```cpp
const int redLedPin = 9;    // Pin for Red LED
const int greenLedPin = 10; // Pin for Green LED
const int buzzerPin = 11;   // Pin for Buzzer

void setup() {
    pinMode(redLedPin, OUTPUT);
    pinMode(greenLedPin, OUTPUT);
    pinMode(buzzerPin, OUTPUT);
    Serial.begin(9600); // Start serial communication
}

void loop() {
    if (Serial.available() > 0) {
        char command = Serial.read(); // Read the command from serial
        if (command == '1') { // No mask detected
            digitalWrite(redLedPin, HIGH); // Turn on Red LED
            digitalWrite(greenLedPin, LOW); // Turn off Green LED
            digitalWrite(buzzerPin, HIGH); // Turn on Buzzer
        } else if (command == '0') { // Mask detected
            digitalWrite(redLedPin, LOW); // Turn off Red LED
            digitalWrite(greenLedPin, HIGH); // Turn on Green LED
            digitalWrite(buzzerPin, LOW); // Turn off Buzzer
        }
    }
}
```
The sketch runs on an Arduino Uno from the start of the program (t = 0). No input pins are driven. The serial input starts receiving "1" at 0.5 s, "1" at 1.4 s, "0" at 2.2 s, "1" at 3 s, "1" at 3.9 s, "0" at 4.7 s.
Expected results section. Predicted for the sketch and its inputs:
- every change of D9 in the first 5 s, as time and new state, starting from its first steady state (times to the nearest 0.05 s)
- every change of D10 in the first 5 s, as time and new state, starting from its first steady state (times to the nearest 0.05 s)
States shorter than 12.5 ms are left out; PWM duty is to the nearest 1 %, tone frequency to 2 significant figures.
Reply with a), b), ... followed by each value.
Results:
a) 0 s low; 0.5 s high; 2.2 s low; 3 s high; 4.7 s low
b) 0 s low; 2.2 s high; 3 s low; 4.7 s high
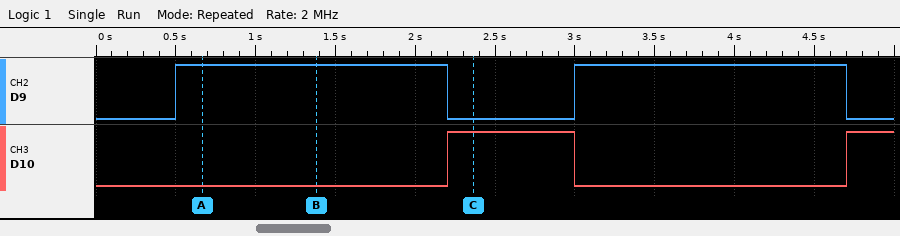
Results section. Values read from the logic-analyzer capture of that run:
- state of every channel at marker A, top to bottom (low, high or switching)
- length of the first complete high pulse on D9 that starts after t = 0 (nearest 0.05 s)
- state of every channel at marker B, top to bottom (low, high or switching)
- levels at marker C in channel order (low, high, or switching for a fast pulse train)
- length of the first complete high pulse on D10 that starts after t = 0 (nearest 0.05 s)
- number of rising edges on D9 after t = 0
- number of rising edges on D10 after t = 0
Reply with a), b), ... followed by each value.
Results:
a) D9 high, D10 low
b) 1.70 s
c) D9 high, D10 low
d) D9 low, D10 high
e) 0.80 s
f) 2
g) 2
